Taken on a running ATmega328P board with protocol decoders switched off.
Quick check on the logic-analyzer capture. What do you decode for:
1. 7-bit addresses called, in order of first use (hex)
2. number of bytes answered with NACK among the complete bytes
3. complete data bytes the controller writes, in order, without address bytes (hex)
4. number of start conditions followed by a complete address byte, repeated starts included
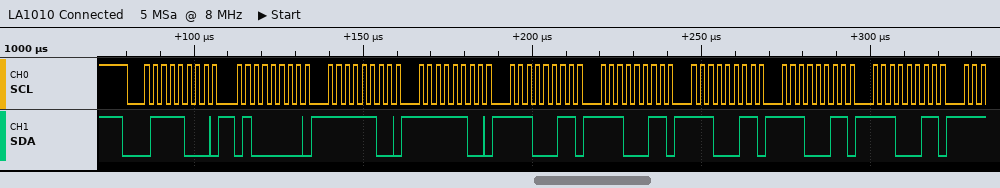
0x3C
0
40 FC FC E3 E3 E3 E3 E3
1
